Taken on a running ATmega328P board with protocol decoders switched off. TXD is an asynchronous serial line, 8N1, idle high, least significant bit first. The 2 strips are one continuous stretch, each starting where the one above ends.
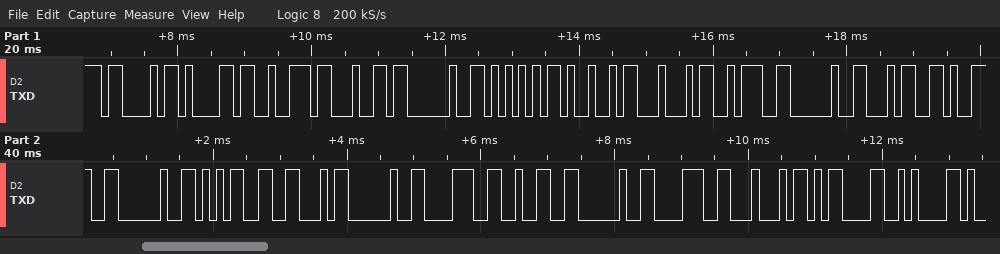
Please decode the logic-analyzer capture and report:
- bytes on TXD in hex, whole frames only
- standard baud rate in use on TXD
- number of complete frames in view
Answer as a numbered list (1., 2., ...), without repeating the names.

1. 43 61 72 64 20 55 49 44 3A 20 34 39 20 35 46 20 38 32 20 38 44 0D 0A
2. 9600 baud
3. 23
